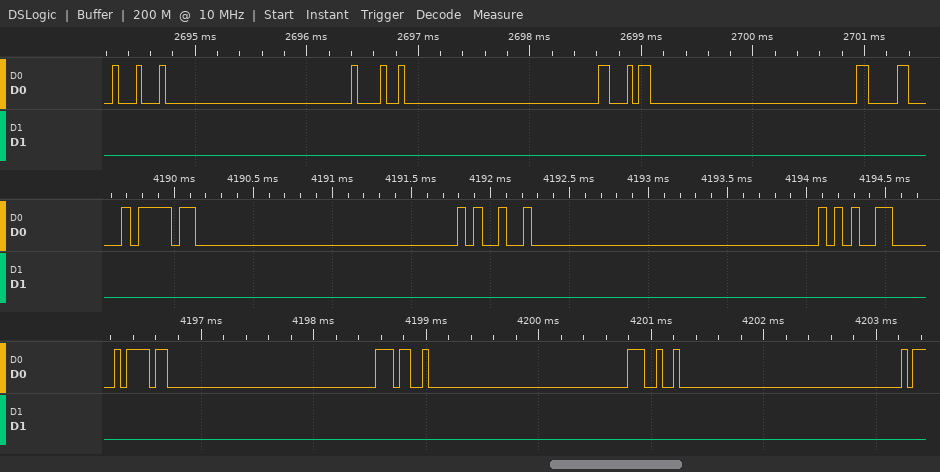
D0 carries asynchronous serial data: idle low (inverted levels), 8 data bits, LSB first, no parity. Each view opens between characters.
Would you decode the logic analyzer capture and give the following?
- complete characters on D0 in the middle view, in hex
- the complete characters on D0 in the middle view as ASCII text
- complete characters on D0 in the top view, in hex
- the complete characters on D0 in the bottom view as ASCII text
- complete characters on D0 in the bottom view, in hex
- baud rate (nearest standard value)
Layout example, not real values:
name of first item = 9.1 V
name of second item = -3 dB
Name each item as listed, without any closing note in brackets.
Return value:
complete characters on D0 in the middle view, in hex = 21, 6D, 35
the complete characters on D0 in the middle view as ASCII text = "!m5"
complete characters on D0 in the top view, in hex = 77, 6F, 2E, 3E
the complete characters on D0 in the bottom view as ASCII text = "!dl"
complete characters on D0 in the bottom view, in hex = 21, 64, 6C
baud rate = 19200 baud
